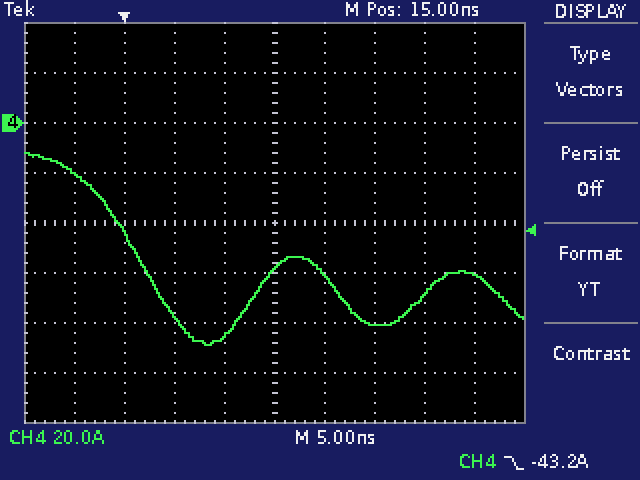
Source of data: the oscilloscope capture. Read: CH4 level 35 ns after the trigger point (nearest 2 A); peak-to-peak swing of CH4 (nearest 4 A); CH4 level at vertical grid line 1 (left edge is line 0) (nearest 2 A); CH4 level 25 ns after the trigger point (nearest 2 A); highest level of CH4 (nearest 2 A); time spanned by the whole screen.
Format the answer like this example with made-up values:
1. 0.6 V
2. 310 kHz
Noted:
1. -60 A
2. 76 A
3. -20 A
4. -80 A
5. -12 A
6. 50 ns
